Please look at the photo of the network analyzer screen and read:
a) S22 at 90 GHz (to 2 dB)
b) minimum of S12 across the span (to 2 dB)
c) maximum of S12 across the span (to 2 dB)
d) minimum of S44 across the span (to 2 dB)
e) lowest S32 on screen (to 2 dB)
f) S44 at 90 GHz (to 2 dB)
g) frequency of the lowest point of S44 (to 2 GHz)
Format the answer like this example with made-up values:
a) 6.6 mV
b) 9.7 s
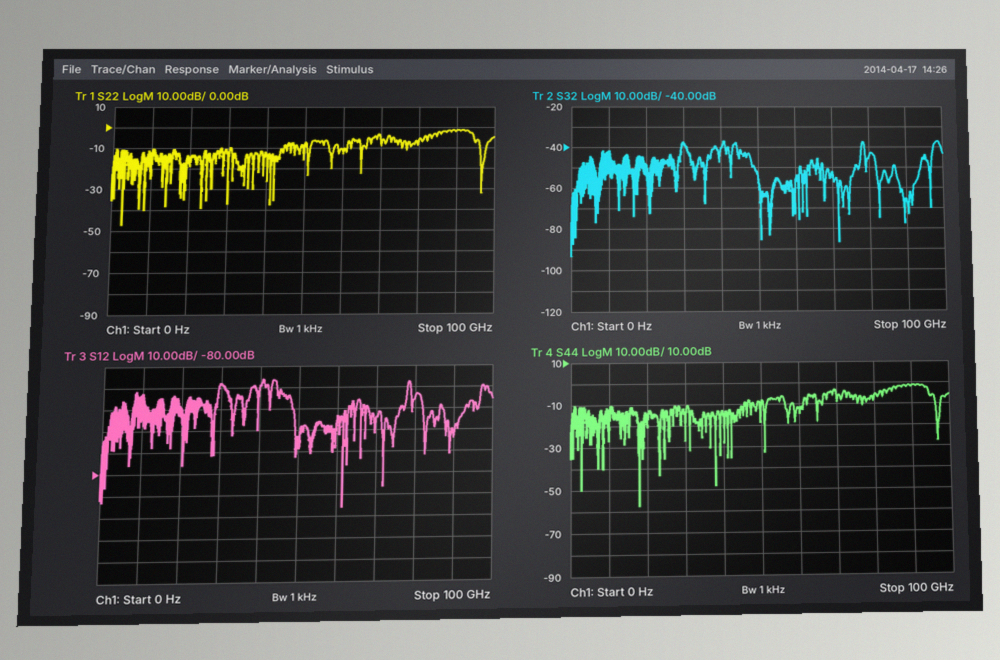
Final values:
a) -2 dB
b) -96 dB
c) -36 dB
d) -58 dB
e) -94 dB
f) -2 dB
g) 18 GHz
